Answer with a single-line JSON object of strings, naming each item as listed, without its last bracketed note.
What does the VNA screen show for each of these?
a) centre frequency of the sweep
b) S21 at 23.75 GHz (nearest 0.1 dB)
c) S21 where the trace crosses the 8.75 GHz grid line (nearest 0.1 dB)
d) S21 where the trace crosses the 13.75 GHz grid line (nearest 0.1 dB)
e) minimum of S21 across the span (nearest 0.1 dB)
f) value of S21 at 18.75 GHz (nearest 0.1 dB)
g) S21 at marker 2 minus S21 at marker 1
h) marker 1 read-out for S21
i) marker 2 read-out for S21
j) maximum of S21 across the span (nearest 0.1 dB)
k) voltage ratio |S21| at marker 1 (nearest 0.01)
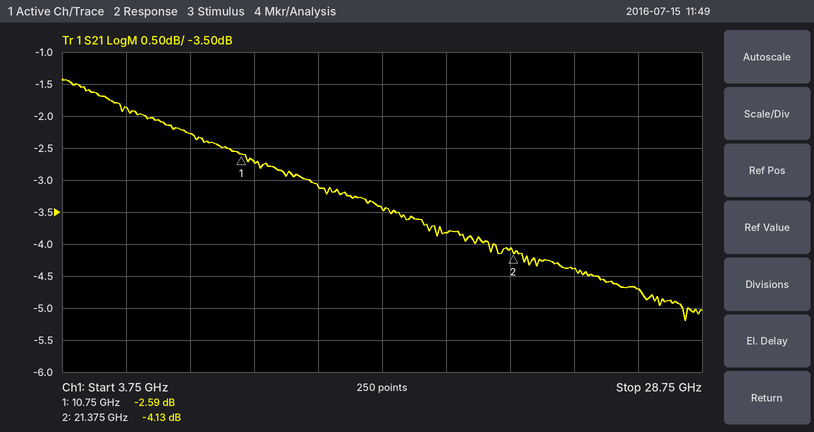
{"centre frequency of the sweep": "16.25 GHz", "S21 at 23.75 GHz": "-4.4 dB", "S21 where the trace crosses the 8.75 GHz grid line": "-2.3 dB", "S21 where the trace crosses the 13.75 GHz grid line": "-3.1 dB", "minimum of S21 across the span": "-5.2 dB", "value of S21 at 18.75 GHz": "-3.8 dB", "S21 at marker 2 minus S21 at marker 1": "-1.54 dB", "marker 1 read-out for S21": "-2.59 dB", "marker 2 read-out for S21": "-4.13 dB", "maximum of S21 across the span": "-1.4 dB", "voltage ratio |S21| at marker 1": "0.74"}
